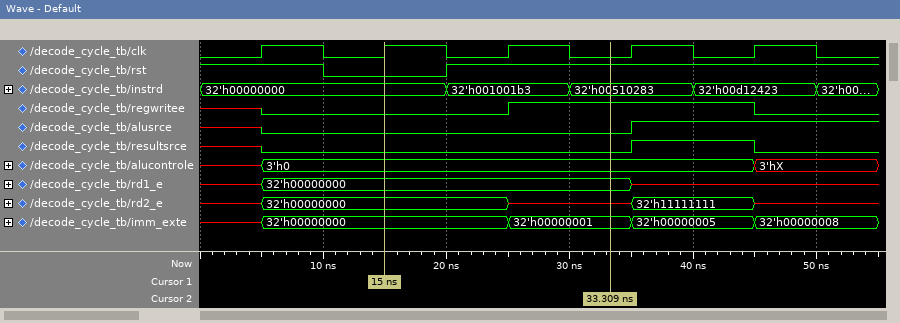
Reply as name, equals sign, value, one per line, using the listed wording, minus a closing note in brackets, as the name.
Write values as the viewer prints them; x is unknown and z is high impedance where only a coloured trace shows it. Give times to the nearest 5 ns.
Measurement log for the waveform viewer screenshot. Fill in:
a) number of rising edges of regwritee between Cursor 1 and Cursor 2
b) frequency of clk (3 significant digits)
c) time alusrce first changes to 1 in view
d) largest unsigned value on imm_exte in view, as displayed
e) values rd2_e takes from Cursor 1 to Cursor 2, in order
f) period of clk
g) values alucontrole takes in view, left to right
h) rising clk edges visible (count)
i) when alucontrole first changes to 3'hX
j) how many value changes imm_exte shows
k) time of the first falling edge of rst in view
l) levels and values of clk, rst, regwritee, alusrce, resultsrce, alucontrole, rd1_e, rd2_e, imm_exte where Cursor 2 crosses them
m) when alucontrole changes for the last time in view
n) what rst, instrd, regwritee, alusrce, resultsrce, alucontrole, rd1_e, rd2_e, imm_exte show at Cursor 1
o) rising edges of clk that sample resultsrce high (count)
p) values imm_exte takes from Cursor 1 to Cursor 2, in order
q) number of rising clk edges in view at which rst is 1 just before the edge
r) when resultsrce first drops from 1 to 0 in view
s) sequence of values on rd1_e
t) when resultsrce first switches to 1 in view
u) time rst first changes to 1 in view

number of rising edges of regwritee between Cursor 1 and Cursor 2 = 1
frequency of clk = 100 MHz
time alusrce first changes to 1 in view = 35 ns
largest unsigned value on imm_exte in view, as displayed = 32'h00000008
values rd2_e takes from Cursor 1 to Cursor 2, in order = 32'h00000000, x
period of clk = 10 ns
values alucontrole takes in view, left to right = x, 3'h0, 3'hX
rising clk edges visible = 5
when alucontrole first changes to 3'hX = 45 ns
how many value changes imm_exte shows = 4
time of the first falling edge of rst in view = 10 ns
levels and values of clk, rst, regwritee, alusrce, resultsrce, alucontrole, rd1_e, rd2_e, imm_exte where Cursor 2 crosses them = clk=0, rst=1, regwritee=1, alusrce=0, resultsrce=0, alucontrole=3'h0, rd1_e=32'h00000000, rd2_e=x, imm_exte=32'h00000001
when alucontrole changes for the last time in view = 45 ns
what rst, instrd, regwritee, alusrce, resultsrce, alucontrole, rd1_e, rd2_e, imm_exte show at Cursor 1 = rst=0, instrd=32'h00000000, regwritee=0, alusrce=0, resultsrce=0, alucontrole=3'h0, rd1_e=32'h00000000, rd2_e=32'h00000000, imm_exte=32'h00000000
rising edges of clk that sample resultsrce high = 1
values imm_exte takes from Cursor 1 to Cursor 2, in order = 32'h00000000, 32'h00000001
number of rising clk edges in view at which rst is 1 just before the edge = 4
when resultsrce first drops from 1 to 0 in view = 45 ns
sequence of values on rd1_e = x, 32'h00000000, x
when resultsrce first switches to 1 in view = 35 ns
time rst first changes to 1 in view = 20 ns
